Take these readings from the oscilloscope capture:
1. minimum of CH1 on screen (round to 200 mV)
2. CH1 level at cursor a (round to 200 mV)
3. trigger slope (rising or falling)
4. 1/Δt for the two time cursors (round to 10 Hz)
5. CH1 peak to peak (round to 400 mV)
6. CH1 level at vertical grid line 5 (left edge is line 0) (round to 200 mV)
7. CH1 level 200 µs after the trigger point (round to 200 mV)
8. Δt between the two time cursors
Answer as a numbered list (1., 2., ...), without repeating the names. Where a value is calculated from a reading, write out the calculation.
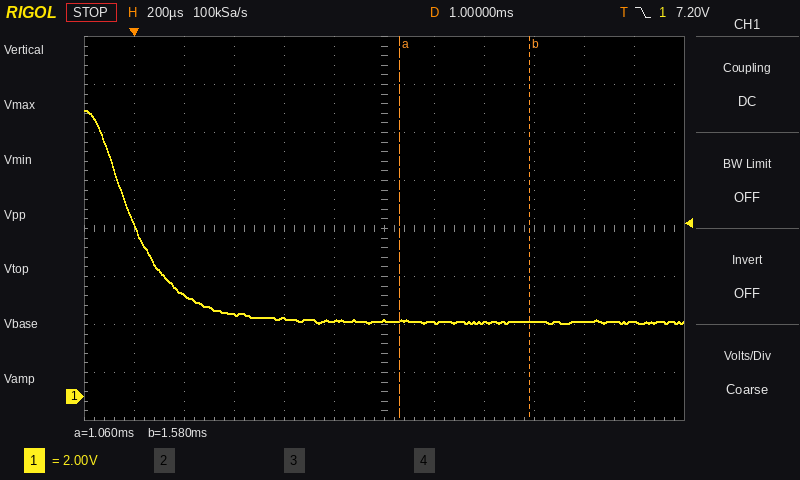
1. 3.0 V
2. 3.2 V
3. falling
4. 1 / 520 µs ≈ 1.92 kHz
5. 8.8 V
6. 3.2 V
7. 4.2 V
8. 1.58 ms − (1.06 ms) = 520 µs
